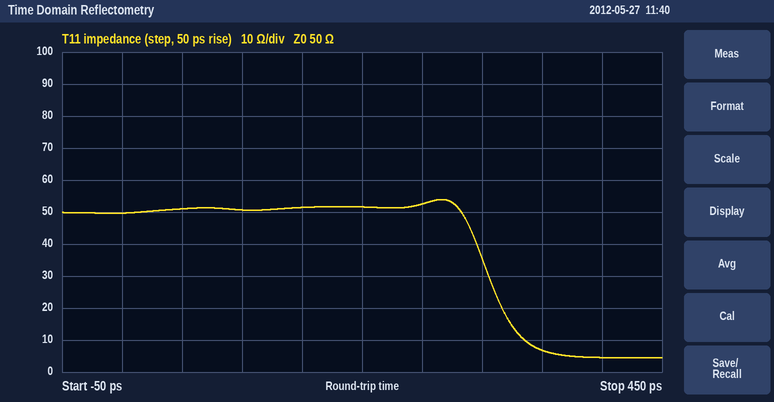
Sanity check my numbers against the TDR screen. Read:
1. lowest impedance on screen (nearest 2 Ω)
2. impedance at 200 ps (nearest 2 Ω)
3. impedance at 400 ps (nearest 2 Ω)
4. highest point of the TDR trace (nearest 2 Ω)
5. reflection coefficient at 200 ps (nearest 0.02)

4 Ω
52 Ω
4 Ω
54 Ω
+0.02
